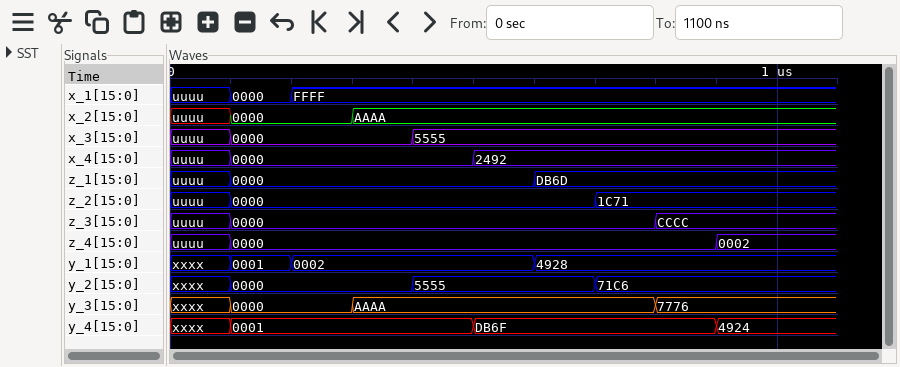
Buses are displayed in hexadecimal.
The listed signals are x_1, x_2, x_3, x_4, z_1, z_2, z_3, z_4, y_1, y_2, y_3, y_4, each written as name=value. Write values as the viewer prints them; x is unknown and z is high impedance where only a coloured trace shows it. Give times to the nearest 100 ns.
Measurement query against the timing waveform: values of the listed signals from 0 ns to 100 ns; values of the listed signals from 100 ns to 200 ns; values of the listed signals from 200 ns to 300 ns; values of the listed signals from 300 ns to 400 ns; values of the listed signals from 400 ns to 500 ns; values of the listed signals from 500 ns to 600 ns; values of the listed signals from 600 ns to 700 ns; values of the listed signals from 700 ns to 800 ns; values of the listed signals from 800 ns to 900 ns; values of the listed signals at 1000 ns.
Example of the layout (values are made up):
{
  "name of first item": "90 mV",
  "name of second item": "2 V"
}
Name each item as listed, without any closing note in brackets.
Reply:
{
  "values of the listed signals from 0 ns to 100 ns": "x_1=uuuu, x_2=uuuu, x_3=uuuu, x_4=uuuu, z_1=uuuu, z_2=uuuu, z_3=uuuu, z_4=uuuu, y_1=xxxx, y_2=xxxx, y_3=xxxx, y_4=xxxx",
  "values of the listed signals from 100 ns to 200 ns": "x_1=0000, x_2=0000, x_3=0000, x_4=0000, z_1=0000, z_2=0000, z_3=0000, z_4=0000, y_1=0001, y_2=0000, y_3=0000, y_4=0001",
  "values of the listed signals from 200 ns to 300 ns": "x_1=FFFF, x_2=0000, x_3=0000, x_4=0000, z_1=0000, z_2=0000, z_3=0000, z_4=0000, y_1=0002, y_2=0000, y_3=0000, y_4=0001",
  "values of the listed signals from 300 ns to 400 ns": "x_1=FFFF, x_2=AAAA, x_3=0000, x_4=0000, z_1=0000, z_2=0000, z_3=0000, z_4=0000, y_1=0002, y_2=0000, y_3=AAAA, y_4=0001",
  "values of the listed signals from 400 ns to 500 ns": "x_1=FFFF, x_2=AAAA, x_3=5555, x_4=0000, z_1=0000, z_2=0000, z_3=0000, z_4=0000, y_1=0002, y_2=5555, y_3=AAAA, y_4=0001",
  "values of the listed signals from 500 ns to 600 ns": "x_1=FFFF, x_2=AAAA, x_3=5555, x_4=2492, z_1=0000, z_2=0000, z_3=0000, z_4=0000, y_1=0002, y_2=5555, y_3=AAAA, y_4=DB6F",
  "values of the listed signals from 600 ns to 700 ns": "x_1=FFFF, x_2=AAAA, x_3=5555, x_4=2492, z_1=DB6D, z_2=0000, z_3=0000, z_4=0000, y_1=4928, y_2=5555, y_3=AAAA, y_4=DB6F",
  "values of the listed signals from 700 ns to 800 ns": "x_1=FFFF, x_2=AAAA, x_3=5555, x_4=2492, z_1=DB6D, z_2=1C71, z_3=0000, z_4=0000, y_1=4928, y_2=71C6, y_3=AAAA, y_4=DB6F",
  "values of the listed signals from 800 ns to 900 ns": "x_1=FFFF, x_2=AAAA, x_3=5555, x_4=2492, z_1=DB6D, z_2=1C71, z_3=CCCC, z_4=0000, y_1=4928, y_2=71C6, y_3=7776, y_4=DB6F",
  "values of the listed signals at 1000 ns": "x_1=FFFF, x_2=AAAA, x_3=5555, x_4=2492, z_1=DB6D, z_2=1C71, z_3=CCCC, z_4=0002, y_1=4928, y_2=71C6, y_3=7776, y_4=4924"
}
